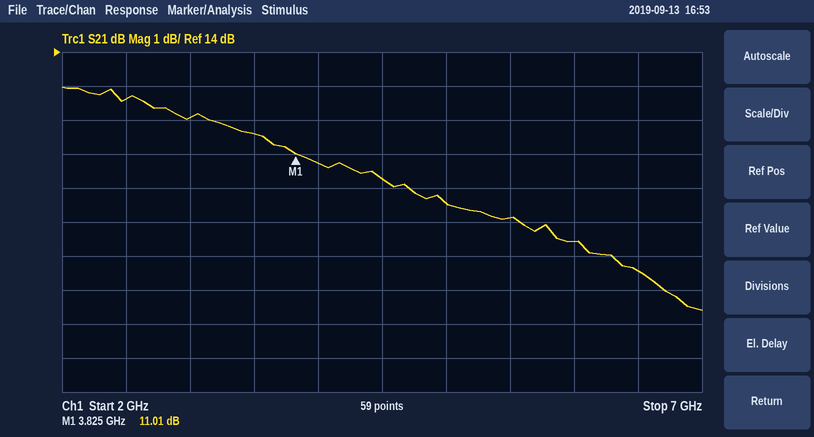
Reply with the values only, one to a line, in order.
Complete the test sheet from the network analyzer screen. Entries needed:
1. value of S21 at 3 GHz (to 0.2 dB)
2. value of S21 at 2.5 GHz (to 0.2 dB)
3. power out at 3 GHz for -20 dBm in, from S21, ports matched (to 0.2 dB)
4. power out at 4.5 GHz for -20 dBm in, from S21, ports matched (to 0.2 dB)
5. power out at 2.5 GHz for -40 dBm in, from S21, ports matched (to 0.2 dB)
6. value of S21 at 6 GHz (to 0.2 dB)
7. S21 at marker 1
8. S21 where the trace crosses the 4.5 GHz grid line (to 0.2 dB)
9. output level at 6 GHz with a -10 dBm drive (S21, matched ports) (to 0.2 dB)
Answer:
12.0 dB
12.6 dB
-8.0 dBm
-9.8 dBm
-27.4 dBm
8.4 dB
11.01 dB
10.2 dB
-1.6 dBm
